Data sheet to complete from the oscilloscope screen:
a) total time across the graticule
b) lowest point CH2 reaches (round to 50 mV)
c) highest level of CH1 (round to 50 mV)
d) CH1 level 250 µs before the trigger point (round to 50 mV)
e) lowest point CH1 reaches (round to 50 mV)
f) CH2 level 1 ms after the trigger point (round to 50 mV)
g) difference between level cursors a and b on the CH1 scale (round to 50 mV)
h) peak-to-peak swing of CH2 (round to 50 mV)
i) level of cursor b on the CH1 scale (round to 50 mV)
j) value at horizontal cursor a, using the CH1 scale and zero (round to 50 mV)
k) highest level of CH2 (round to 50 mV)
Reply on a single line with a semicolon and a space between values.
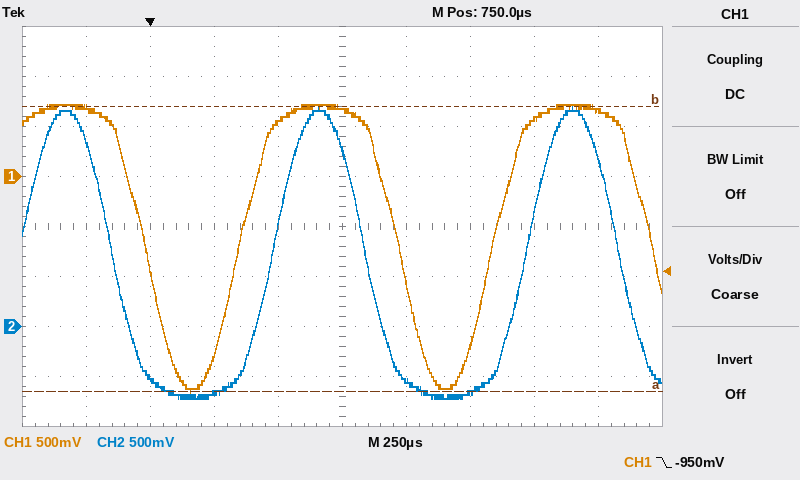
2.5 ms; -700 mV; 700 mV; 700 mV; -2.15 V; -550 mV; 2.85 V; 2.90 V; 700 mV; -2.15 V; 2.20 V
